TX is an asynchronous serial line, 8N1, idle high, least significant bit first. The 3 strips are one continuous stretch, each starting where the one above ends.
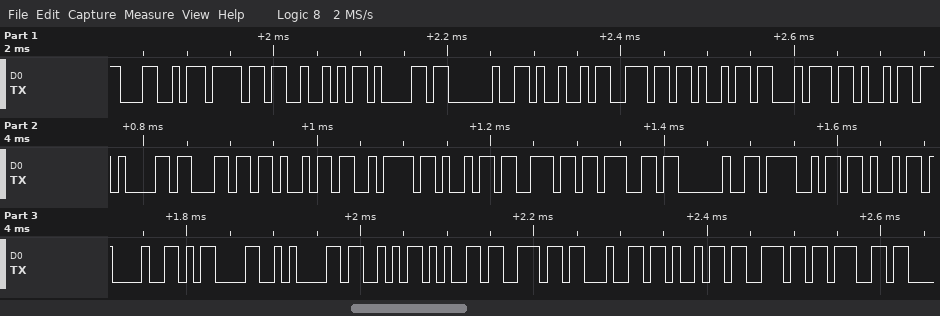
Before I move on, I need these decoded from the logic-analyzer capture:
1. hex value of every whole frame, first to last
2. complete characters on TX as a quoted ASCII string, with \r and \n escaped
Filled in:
4C 6F 52 61 20 49 6E 69 74 69 61 6C 69 7A 69 6E 67 20 4F 4B 21 0D 0A 53 65 6E 64 69 6E 67
"LoRa Initializing OK!\r\nSending"
